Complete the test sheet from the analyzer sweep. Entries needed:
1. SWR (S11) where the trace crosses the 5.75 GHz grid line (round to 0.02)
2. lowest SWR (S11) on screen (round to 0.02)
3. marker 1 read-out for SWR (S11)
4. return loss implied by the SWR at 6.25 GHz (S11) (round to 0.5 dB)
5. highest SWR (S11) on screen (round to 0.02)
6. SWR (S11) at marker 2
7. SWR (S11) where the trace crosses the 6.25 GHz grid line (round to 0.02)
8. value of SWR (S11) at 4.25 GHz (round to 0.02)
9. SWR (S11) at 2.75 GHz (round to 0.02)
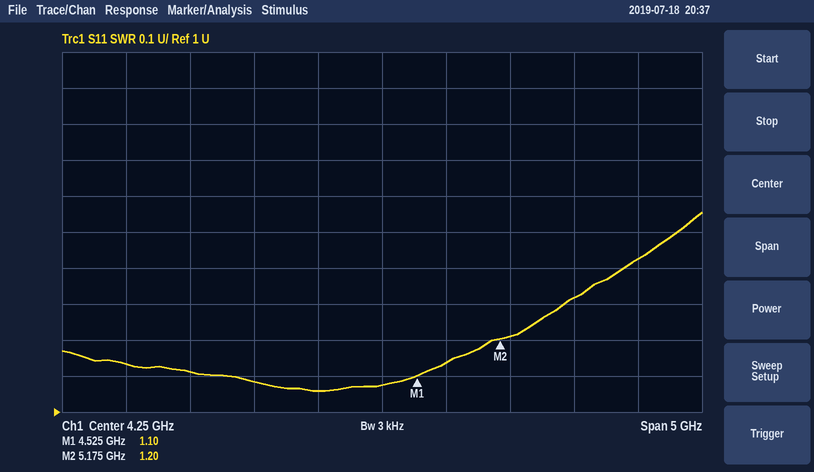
1.32
1.06
1.10
15.0 dB
1.56
1.20
1.42
1.08
1.12
